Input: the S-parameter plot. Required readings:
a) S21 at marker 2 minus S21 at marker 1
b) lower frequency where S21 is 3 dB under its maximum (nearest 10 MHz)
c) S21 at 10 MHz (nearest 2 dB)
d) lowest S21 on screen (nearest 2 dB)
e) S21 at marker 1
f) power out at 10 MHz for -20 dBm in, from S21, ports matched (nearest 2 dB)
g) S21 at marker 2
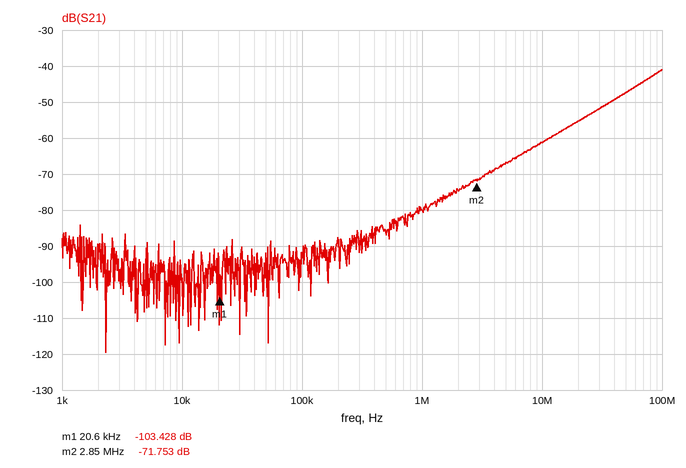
31.675 dB
70 MHz
-62 dB
-120 dB
-103.428 dB
-82 dBm
-71.753 dB
